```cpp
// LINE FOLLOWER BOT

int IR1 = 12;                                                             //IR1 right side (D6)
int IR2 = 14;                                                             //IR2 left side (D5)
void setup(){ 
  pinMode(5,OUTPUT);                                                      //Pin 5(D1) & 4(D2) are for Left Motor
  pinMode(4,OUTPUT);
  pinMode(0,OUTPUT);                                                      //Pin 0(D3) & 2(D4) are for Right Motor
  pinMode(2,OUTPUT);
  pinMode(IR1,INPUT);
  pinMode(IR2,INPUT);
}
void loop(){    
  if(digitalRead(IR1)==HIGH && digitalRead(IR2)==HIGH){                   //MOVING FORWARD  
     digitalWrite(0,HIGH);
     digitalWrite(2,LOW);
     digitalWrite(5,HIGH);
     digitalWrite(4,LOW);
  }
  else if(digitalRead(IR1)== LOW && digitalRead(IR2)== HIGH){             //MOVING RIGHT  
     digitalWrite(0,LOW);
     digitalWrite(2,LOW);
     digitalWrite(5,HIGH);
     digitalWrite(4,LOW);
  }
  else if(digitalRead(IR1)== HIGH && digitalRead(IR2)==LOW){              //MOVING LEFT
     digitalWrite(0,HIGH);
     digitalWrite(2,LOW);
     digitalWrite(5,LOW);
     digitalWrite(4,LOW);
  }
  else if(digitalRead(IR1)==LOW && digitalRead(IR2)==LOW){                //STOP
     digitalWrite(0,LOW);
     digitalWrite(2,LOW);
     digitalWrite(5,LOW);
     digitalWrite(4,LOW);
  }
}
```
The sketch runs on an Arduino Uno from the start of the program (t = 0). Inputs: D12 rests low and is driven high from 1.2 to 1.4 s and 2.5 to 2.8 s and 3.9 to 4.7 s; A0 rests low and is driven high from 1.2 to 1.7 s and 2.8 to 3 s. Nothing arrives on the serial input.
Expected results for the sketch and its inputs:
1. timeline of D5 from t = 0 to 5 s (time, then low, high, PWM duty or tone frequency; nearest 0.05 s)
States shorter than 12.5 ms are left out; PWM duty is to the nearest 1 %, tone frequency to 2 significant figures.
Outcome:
0 s low; 1.2 s high; 1.7 s low; 2.8 s high; 3 s low
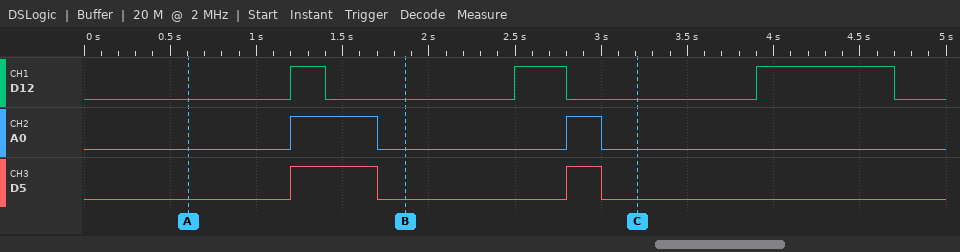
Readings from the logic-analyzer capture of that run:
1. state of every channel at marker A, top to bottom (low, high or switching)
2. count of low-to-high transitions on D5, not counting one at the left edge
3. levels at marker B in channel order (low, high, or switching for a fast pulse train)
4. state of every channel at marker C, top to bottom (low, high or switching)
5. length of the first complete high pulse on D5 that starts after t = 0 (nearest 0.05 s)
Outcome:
D12 low, A0 low, D5 low
2
D12 low, A0 low, D5 low
D12 low, A0 low, D5 low
0.50 s
